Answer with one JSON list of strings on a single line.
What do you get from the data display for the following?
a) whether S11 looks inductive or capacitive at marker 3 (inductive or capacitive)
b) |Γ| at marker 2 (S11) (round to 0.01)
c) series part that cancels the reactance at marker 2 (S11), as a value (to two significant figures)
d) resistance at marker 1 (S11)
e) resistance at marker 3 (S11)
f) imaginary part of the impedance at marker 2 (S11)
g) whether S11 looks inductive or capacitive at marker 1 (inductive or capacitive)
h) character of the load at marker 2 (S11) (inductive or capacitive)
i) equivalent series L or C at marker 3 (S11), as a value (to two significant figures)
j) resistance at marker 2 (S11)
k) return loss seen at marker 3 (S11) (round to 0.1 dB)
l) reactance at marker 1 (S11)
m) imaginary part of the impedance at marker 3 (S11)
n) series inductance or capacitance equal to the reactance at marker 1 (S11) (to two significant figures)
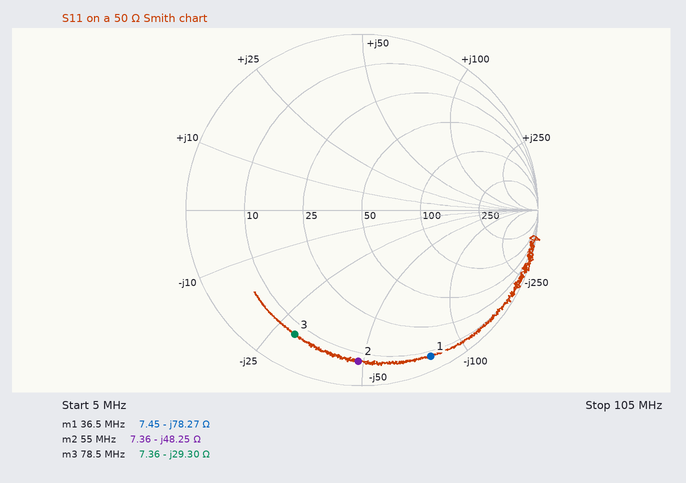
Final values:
["capacitive", "0.86", "140 nH", "7.45 Ω", "7.36 Ω", "-48.25 Ω", "capacitive", "capacitive", "69 pF", "7.36 Ω", "1.9 dB", "-78.27 Ω", "-29.30 Ω", "56 pF"]
